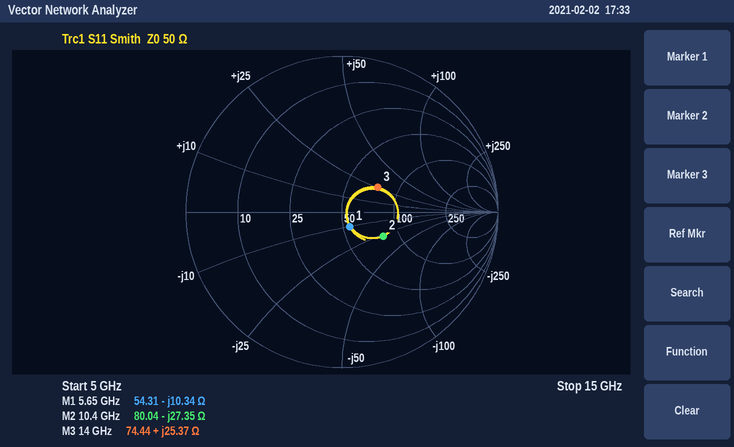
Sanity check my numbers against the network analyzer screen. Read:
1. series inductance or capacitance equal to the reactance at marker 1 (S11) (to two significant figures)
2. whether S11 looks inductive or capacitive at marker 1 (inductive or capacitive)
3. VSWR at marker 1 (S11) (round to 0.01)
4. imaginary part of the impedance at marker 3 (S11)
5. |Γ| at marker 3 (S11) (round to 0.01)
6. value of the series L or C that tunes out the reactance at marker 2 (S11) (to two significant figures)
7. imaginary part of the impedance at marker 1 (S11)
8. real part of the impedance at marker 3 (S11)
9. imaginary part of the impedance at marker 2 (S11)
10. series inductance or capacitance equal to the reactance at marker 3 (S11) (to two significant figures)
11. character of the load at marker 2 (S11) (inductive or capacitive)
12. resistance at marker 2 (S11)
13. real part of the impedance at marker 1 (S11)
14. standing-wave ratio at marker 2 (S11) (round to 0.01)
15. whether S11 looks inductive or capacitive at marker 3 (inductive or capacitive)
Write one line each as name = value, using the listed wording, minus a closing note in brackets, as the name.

series inductance or capacitance equal to the reactance at marker 1 (S11) = 2.7 pF
whether S11 looks inductive or capacitive at marker 1 = capacitive
VSWR at marker 1 (S11) = 1.24
imaginary part of the impedance at marker 3 = +25.37 Ω
|Γ| at marker 3 (S11) = 0.28
value of the series L or C that tunes out the reactance at marker 2 (S11) = 420 pH
imaginary part of the impedance at marker 1 = -10.34 Ω
real part of the impedance at marker 3 = 74.44 Ω
imaginary part of the impedance at marker 2 = -27.35 Ω
series inductance or capacitance equal to the reactance at marker 3 (S11) = 290 pH
character of the load at marker 2 (S11) = capacitive
resistance at marker 2 = 80.04 Ω
real part of the impedance at marker 1 = 54.31 Ω
standing-wave ratio at marker 2 (S11) = 1.88
whether S11 looks inductive or capacitive at marker 3 = inductive
